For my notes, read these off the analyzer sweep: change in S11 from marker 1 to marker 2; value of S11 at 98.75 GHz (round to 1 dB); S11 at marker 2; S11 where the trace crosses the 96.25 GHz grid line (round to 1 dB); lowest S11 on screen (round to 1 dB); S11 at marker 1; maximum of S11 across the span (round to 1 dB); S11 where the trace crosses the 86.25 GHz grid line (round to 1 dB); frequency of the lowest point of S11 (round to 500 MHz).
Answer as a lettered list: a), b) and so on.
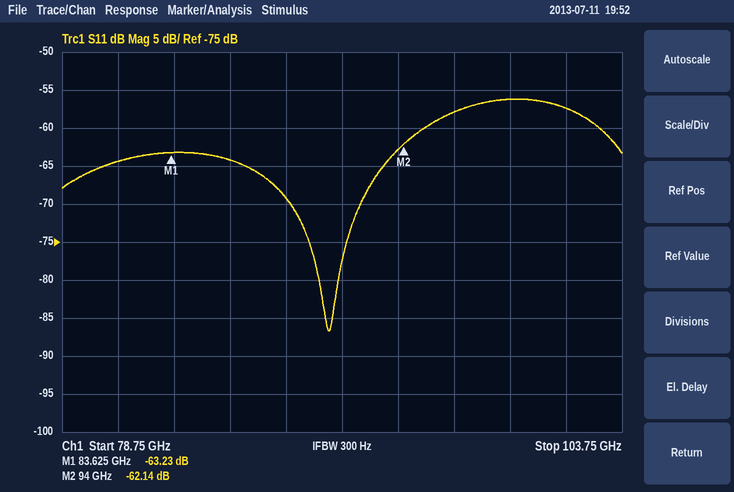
a) 1.09 dB
b) -56 dB
c) -62.14 dB
d) -58 dB
e) -87 dB
f) -63.23 dB
g) -56 dB
h) -64 dB
i) 90.5 GHz
